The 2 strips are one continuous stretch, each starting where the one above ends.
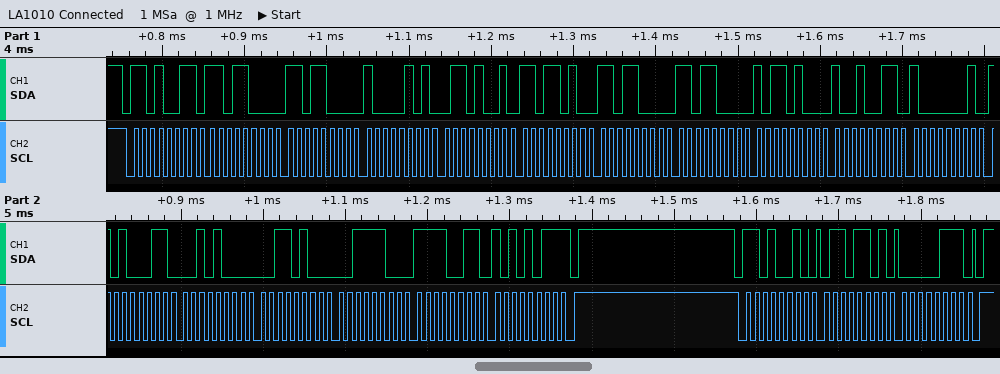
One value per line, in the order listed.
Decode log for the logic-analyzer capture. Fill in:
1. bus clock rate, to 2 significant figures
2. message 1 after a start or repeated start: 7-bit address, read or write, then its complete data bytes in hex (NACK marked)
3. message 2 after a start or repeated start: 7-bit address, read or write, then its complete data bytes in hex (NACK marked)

100 kHz
0x69 read: D8 D8 85 69 DA D8 D8 B4 93 81 A3 28 34 3C F3 AB NACK
0x69 write: 6D 07
